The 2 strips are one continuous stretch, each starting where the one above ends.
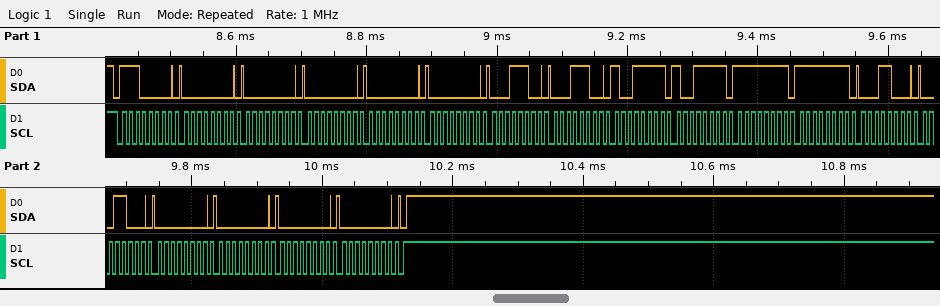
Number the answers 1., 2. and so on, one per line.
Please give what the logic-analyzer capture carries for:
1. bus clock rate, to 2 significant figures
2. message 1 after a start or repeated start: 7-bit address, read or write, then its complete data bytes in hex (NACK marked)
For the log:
1. 100 kHz
2. 0x70 write: 00 00 00 00 00 1C 1C 9F 9F FF FF 18 18 00 00 00 00
